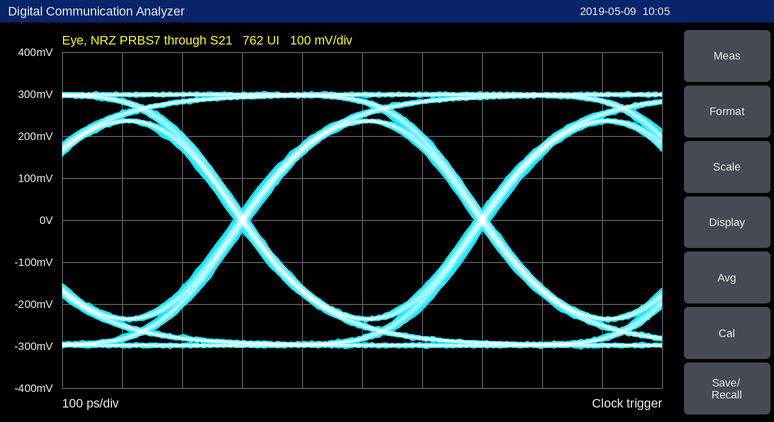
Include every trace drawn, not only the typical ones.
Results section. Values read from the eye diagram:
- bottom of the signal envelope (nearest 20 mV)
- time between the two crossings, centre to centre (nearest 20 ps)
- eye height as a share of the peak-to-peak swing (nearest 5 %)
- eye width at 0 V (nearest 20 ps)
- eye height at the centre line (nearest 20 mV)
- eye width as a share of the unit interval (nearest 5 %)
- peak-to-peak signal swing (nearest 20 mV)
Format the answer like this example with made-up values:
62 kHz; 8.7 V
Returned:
-300 mV; 400 ps; 75 %; 380 ps; 460 mV; 95 %; 620 mV
